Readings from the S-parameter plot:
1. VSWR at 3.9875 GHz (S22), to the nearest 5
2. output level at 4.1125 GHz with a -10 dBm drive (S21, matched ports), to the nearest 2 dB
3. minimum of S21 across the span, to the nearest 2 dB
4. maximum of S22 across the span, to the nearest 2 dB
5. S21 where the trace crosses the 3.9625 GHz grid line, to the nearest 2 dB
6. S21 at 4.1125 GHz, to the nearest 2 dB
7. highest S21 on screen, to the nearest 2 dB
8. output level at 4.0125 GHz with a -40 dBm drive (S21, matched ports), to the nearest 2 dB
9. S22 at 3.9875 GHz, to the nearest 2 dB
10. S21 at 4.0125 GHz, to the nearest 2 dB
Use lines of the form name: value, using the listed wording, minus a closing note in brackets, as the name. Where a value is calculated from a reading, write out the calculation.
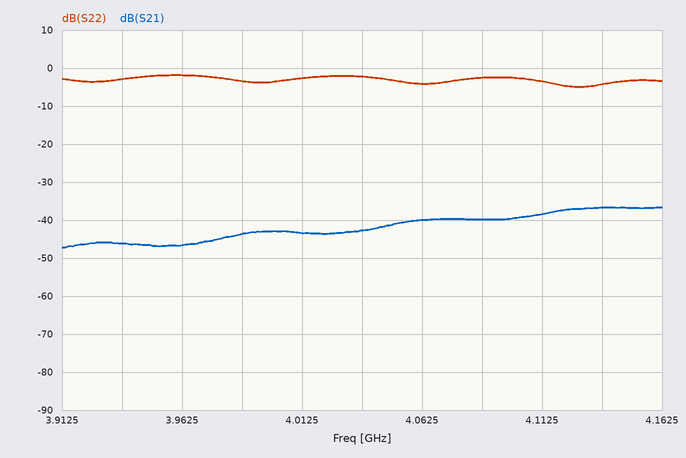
VSWR at 3.9875 GHz (S22), to the nearest 5: |Γ| = 10^(-4/20) = 0.6310; VSWR = (1 + 0.6310)/(1 − 0.6310) ≈ 4.42, so 5 to the nearest 5
output level at 4.1125 GHz with a -10 dBm drive (S21, matched ports), to the nearest 2 dB: -10 dBm + (-38 dB) = -48 dBm
minimum of S21 across the span, to the nearest 2 dB: -48 dB
maximum of S22 across the span, to the nearest 2 dB: -2 dB
S21 where the trace crosses the 3.9625 GHz grid line, to the nearest 2 dB: -46 dB
S21 at 4.1125 GHz, to the nearest 2 dB: -38 dB
highest S21 on screen, to the nearest 2 dB: -36 dB
output level at 4.0125 GHz with a -40 dBm drive (S21, matched ports), to the nearest 2 dB: -40 dBm + (-44 dB) = -84 dBm
S22 at 3.9875 GHz, to the nearest 2 dB: -4 dB
S21 at 4.0125 GHz, to the nearest 2 dB: -44 dB
